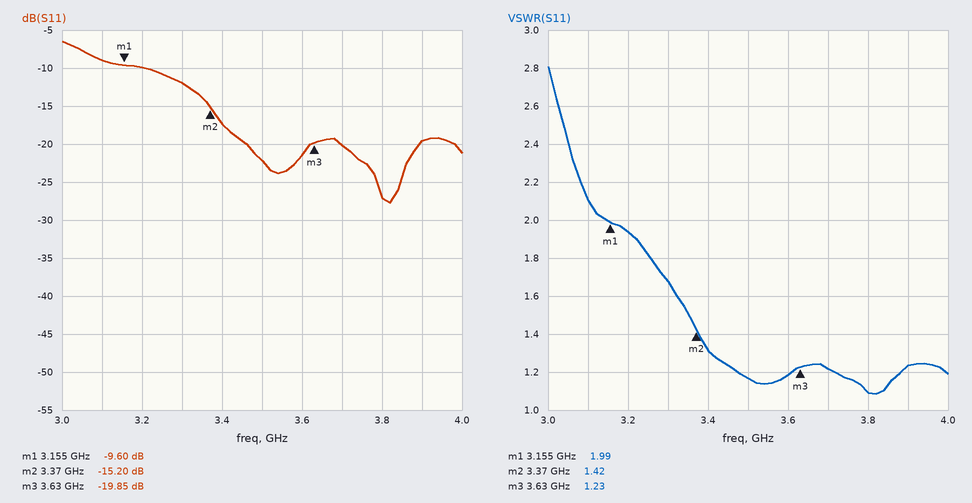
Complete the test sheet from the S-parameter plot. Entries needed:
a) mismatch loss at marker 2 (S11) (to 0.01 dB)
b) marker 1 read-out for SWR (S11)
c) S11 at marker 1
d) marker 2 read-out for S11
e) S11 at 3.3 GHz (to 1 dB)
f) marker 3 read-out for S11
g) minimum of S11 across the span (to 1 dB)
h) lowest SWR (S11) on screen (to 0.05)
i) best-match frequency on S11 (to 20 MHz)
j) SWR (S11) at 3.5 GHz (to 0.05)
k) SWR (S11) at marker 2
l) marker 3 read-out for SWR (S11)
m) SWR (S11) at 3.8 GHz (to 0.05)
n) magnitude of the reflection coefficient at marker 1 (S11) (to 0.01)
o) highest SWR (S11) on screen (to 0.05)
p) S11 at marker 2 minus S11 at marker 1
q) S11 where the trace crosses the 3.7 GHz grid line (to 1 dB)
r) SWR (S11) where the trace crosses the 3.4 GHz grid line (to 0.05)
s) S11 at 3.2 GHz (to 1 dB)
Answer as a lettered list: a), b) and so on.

a) 0.13 dB
b) 1.99
c) -9.60 dB
d) -15.20 dB
e) -12 dB
f) -19.85 dB
g) -28 dB
h) 1.10
i) 3.82 GHz
j) 1.15
k) 1.42
l) 1.23
m) 1.10
n) 0.33
o) 2.80
p) -5.60 dB
q) -20 dB
r) 1.30
s) -10 dB
